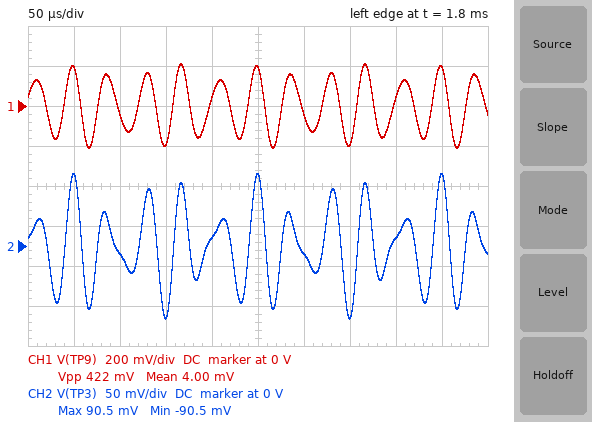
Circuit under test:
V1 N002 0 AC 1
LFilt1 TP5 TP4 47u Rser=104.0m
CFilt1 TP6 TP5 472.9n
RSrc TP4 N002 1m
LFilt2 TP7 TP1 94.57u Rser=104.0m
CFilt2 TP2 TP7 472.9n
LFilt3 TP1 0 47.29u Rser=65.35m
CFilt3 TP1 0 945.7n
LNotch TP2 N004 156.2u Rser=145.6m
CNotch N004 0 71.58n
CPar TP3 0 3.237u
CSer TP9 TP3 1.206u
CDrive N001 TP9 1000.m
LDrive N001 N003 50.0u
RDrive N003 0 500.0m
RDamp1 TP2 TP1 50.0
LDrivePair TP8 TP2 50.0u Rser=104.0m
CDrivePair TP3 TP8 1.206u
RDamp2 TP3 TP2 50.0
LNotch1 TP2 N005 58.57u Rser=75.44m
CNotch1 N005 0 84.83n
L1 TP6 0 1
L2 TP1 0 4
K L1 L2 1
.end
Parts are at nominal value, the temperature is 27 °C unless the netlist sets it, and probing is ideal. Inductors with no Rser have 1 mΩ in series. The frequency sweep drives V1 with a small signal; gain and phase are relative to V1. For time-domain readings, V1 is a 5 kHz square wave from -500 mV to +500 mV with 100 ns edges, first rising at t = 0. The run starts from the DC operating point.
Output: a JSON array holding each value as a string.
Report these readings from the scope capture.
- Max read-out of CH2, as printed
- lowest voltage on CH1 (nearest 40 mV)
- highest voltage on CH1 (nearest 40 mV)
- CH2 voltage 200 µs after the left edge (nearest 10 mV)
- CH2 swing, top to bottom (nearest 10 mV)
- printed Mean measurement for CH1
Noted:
["90.5 mV", "-200 mV", "200 mV", "10 mV", "180 mV", "4.00 mV"]
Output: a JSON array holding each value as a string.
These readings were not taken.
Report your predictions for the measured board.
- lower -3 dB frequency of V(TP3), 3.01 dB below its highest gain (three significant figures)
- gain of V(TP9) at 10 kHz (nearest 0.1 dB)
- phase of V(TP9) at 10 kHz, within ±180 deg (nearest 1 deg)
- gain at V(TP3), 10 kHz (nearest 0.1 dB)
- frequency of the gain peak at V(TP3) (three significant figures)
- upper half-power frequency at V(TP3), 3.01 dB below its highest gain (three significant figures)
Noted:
["28.4 kHz", "-55.1 dB", "-39 deg", "-45.1 dB", "28.9 kHz", "29.4 kHz"]
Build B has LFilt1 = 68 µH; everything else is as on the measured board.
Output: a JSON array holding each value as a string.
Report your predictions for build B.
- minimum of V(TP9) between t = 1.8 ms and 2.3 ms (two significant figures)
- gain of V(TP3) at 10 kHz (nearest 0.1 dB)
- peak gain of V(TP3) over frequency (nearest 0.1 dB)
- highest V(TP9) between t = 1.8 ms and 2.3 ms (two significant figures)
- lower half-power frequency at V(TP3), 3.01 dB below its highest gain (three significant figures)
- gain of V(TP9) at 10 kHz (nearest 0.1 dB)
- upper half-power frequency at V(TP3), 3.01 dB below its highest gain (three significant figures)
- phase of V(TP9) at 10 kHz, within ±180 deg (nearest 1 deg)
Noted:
["-420 mV", "-44.7 dB", "12.3 dB", "420 mV", "26.6 kHz", "-54.7 dB", "27.2 kHz", "-39 deg"]
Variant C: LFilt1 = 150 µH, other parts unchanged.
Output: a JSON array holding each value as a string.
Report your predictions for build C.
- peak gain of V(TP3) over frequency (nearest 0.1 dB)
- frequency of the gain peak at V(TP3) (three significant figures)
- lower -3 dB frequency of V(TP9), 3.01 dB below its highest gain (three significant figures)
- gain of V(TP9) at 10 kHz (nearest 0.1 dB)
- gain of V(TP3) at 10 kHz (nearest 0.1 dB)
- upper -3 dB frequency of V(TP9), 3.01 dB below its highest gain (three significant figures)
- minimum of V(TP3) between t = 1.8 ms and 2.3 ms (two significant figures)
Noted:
["-5.1 dB", "19.9 kHz", "19.8 kHz", "-53.0 dB", "-43.0 dB", "20.2 kHz", "-57 mV"]
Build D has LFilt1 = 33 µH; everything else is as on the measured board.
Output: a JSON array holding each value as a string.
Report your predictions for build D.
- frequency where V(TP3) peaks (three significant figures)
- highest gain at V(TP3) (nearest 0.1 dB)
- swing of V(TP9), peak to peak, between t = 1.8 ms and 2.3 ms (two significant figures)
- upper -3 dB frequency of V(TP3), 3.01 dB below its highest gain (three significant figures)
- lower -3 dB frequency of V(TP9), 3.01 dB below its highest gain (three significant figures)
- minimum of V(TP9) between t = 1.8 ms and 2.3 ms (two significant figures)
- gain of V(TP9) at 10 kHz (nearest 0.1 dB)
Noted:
["29.7 kHz", "2.0 dB", "330 mV", "30.3 kHz", "29.0 kHz", "-160 mV", "-55.4 dB"]
